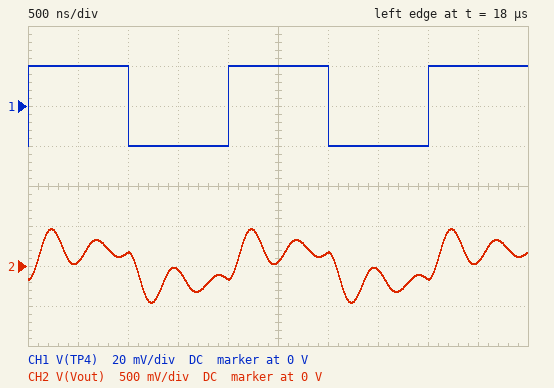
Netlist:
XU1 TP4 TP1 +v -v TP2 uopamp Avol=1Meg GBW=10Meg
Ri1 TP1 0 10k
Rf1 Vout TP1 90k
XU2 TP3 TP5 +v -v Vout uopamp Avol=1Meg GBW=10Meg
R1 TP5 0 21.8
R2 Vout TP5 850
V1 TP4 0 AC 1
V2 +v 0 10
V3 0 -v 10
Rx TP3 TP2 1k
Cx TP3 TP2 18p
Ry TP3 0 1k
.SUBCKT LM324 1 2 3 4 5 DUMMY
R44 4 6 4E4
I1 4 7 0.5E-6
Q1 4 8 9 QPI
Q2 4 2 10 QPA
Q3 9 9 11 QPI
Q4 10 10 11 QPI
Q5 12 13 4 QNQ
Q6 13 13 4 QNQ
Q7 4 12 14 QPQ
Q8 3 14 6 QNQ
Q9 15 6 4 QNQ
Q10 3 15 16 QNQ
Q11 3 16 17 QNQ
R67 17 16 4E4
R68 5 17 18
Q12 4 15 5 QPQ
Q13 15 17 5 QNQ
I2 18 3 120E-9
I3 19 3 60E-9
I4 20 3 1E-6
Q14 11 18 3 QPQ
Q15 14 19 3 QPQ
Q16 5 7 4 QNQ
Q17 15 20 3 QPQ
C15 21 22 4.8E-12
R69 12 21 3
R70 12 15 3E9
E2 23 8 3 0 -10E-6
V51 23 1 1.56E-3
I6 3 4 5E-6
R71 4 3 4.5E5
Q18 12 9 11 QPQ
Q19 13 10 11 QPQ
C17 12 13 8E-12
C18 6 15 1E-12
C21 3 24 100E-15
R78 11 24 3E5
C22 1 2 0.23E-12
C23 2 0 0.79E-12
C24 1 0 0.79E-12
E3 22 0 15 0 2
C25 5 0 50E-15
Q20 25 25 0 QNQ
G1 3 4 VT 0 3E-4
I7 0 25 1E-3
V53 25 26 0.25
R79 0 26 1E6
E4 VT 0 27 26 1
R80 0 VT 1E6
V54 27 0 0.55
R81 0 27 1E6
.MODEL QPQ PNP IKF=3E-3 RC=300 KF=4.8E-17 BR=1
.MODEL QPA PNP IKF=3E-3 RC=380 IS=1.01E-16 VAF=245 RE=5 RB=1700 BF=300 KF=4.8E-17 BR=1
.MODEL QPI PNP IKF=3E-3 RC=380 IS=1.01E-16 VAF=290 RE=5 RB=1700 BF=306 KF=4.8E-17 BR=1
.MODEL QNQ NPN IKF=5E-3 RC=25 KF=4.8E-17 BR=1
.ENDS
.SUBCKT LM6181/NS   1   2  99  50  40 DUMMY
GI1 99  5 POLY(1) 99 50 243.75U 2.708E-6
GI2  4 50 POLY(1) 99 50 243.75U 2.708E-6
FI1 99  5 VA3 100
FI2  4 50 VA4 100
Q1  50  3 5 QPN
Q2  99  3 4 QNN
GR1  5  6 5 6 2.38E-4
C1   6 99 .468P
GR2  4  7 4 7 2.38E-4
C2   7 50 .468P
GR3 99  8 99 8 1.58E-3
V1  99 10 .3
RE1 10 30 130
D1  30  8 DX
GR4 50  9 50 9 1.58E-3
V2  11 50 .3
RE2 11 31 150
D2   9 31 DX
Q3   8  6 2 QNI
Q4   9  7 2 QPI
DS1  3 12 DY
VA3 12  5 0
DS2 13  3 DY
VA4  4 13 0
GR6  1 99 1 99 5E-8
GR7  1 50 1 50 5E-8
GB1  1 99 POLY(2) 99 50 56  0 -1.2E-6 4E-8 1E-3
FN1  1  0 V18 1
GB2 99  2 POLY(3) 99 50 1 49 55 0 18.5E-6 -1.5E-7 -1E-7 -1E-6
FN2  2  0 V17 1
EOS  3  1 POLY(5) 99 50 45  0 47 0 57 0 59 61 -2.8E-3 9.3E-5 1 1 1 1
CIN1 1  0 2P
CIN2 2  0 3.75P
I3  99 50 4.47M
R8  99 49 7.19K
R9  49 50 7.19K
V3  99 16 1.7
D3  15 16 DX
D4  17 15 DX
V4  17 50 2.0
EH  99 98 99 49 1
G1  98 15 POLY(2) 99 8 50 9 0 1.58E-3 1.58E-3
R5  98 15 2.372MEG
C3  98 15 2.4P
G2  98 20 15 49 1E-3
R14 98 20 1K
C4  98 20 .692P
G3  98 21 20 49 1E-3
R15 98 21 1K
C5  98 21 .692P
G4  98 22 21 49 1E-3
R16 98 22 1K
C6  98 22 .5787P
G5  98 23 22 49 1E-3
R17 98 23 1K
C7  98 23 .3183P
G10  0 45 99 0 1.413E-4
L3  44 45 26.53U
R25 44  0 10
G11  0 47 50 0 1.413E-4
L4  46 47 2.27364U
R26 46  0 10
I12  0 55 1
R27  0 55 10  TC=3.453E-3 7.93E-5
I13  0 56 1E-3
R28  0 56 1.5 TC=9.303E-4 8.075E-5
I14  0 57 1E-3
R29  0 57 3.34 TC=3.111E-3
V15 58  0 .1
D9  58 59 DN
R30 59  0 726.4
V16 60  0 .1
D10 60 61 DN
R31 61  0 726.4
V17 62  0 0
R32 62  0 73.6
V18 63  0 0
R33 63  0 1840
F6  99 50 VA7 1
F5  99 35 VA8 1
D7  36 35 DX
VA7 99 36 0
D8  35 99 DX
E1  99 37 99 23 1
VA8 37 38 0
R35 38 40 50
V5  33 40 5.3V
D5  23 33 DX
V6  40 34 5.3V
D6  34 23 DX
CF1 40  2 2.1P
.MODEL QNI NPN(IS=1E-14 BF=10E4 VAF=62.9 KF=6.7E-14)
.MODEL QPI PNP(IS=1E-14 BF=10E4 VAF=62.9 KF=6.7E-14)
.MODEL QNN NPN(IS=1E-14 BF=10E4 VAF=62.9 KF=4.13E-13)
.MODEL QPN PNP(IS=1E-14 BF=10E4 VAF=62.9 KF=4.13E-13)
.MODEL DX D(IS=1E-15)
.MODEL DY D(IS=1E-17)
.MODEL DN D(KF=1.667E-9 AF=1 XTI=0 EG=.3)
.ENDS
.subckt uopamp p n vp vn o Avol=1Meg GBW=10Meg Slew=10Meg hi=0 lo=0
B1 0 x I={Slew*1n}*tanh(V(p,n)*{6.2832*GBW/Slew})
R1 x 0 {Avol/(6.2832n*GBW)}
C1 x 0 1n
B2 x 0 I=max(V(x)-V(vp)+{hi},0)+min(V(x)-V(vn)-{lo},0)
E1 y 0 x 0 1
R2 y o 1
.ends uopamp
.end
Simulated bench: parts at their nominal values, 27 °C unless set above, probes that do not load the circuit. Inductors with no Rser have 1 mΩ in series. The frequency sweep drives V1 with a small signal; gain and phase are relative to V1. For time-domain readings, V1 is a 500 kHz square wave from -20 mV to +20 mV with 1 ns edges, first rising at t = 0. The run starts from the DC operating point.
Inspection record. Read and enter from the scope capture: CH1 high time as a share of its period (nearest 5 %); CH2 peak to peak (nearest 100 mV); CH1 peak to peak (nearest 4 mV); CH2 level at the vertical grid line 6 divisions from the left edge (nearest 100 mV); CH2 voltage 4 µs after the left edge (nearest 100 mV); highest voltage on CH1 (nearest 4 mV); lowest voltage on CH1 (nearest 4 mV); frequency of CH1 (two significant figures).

50 %
900 mV
40 mV
200 mV
-200 mV
20 mV
-20 mV
500 kHz
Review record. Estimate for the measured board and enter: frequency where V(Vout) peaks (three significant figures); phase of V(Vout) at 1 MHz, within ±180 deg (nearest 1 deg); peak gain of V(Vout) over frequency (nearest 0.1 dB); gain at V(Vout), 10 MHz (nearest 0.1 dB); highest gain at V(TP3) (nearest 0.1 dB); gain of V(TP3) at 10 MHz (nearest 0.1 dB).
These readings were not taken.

2.22 MHz
-4 deg
32.7 dB
-3.1 dB
19.8 dB
-3.1 dB
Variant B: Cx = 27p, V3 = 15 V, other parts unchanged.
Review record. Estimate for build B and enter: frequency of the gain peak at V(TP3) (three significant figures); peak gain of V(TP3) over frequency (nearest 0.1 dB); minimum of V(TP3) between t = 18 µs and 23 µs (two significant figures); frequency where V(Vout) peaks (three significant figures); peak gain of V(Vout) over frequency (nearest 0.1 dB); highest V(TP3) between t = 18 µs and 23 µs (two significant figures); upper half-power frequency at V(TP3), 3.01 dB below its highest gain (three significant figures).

2.28 MHz
18.1 dB
-79 mV
2.23 MHz
31.0 dB
79 mV
2.65 MHz
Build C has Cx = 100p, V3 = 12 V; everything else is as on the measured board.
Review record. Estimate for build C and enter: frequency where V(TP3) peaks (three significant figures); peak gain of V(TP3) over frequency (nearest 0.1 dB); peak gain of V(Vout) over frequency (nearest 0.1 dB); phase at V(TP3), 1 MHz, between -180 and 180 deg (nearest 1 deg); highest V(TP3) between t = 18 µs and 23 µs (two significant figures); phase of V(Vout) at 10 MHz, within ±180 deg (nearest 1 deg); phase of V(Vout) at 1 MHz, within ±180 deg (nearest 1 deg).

2.83 MHz
16.4 dB
27.6 dB
70 deg
96 mV
-169 deg
-6 deg
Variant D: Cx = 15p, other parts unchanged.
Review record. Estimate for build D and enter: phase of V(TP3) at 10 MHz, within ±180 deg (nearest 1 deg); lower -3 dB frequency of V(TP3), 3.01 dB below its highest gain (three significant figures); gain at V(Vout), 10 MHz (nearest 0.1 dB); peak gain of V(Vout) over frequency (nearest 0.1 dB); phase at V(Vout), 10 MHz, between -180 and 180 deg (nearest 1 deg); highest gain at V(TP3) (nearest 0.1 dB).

-71 deg
2.02 MHz
-3.6 dB
33.5 dB
-159 deg
20.5 dB
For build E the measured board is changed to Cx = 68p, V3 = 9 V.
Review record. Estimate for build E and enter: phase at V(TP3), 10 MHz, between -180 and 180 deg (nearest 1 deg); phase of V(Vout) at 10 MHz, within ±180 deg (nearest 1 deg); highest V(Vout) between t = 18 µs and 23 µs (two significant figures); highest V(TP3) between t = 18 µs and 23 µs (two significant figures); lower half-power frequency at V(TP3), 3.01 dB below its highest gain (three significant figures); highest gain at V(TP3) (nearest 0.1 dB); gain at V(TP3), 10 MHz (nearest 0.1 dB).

-77 deg
-165 deg
430 mV
91 mV
2.01 MHz
15.6 dB
0.2 dB
